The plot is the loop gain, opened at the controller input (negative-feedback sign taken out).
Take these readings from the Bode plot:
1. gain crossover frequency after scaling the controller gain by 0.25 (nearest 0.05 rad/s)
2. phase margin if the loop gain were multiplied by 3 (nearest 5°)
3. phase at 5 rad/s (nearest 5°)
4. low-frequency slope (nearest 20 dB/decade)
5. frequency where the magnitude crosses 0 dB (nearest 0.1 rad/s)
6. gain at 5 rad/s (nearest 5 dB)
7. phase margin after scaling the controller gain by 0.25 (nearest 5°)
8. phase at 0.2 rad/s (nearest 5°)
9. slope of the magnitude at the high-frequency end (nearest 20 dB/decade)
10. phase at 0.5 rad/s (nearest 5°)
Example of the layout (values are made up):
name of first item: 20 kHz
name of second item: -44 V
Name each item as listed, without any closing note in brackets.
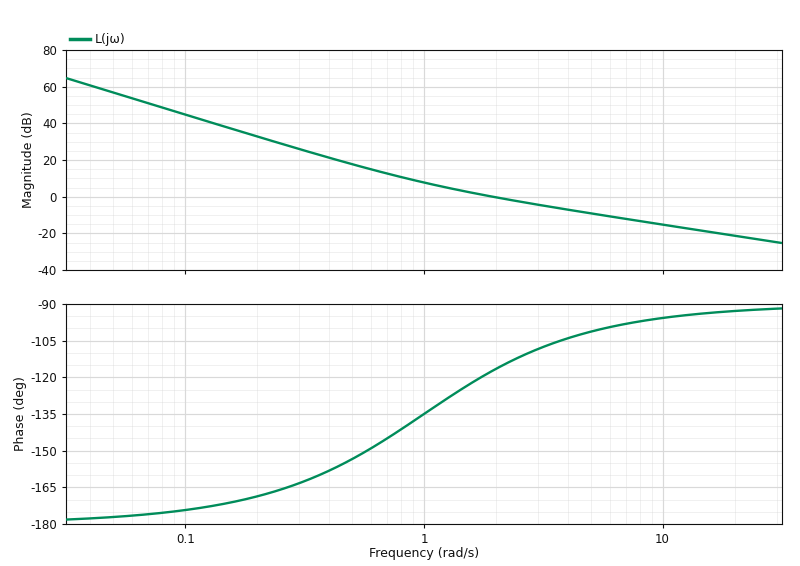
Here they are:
gain crossover frequency after scaling the controller gain by 0.25: 0.75 rad/s
phase margin if the loop gain were multiplied by 3: 80°
phase at 5 rad/s: -100°
low-frequency slope: -40 dB/decade
frequency where the magnitude crosses 0 dB: 1.9 rad/s
gain at 5 rad/s: -10 dB
phase margin after scaling the controller gain by 0.25: 35°
phase at 0.2 rad/s: -170°
slope of the magnitude at the high-frequency end: -20 dB/decade
phase at 0.5 rad/s: -155°
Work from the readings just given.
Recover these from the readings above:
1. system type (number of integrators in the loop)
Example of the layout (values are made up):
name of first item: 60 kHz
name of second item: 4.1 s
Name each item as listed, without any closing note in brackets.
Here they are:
system type: 2
